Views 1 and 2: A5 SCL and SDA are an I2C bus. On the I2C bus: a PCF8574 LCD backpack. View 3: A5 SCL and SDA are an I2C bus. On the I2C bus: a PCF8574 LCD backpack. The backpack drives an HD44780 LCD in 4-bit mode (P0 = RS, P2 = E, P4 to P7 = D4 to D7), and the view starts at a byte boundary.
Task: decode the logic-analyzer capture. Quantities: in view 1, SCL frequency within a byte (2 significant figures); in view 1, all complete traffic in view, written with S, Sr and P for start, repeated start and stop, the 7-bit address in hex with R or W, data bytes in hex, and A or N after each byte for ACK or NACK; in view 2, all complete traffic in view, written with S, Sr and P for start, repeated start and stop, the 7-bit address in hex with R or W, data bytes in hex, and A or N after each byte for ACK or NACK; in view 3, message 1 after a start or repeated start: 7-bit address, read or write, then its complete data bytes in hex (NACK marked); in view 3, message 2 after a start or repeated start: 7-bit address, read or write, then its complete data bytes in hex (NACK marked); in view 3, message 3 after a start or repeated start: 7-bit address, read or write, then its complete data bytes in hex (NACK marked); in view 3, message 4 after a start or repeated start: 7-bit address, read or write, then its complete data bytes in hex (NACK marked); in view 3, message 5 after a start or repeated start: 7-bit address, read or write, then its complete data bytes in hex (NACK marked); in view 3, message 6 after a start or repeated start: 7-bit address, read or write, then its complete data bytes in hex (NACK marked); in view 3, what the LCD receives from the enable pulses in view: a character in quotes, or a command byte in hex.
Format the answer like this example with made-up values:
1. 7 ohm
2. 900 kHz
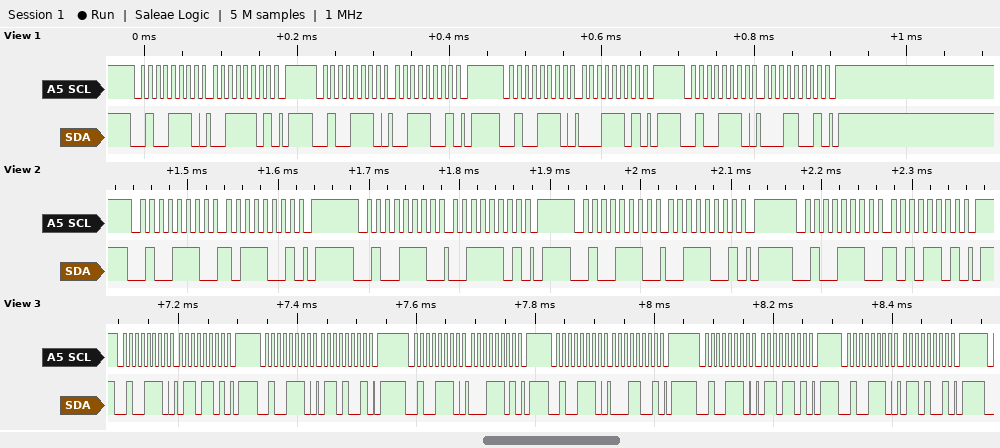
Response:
1. 100 kHz
2. S 27W A 3D A P S 27W A 39 A P S 27W A 1D A P S 27W A 19 A P
3. S 27W A B9 A P S 27W A 3D A P S 27W A 39 A P S 27W A AD A P
4. 0x27 write: 6D
5. 0x27 write: 69
6. 0x27 write: 1D
7. 0x27 write: 19
8. 0x27 write: 6D
9. 0x27 write: 69
10. 'a'
